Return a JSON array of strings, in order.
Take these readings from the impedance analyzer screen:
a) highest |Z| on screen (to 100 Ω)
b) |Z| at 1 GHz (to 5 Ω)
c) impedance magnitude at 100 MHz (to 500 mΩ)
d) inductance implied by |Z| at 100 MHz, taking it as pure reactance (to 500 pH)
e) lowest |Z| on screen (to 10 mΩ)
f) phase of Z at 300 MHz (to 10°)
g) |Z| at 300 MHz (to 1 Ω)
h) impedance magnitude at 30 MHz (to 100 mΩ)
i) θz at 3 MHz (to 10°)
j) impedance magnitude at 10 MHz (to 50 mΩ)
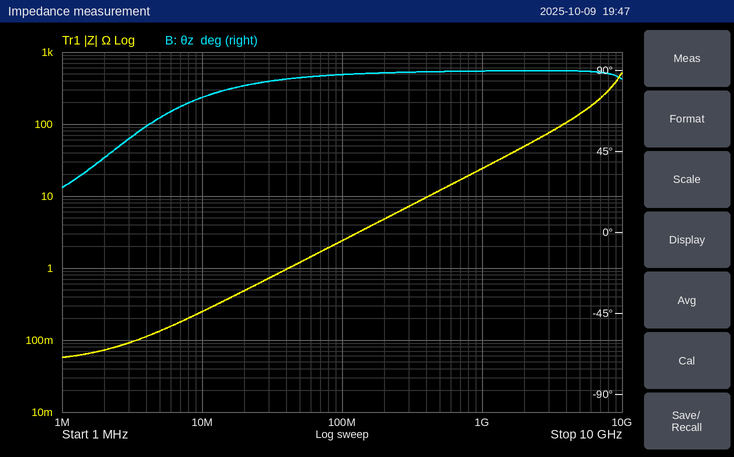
["500 Ω", "25 Ω", "2.5 Ω", "4.0 nH", "60 mΩ", "90°", "7 Ω", "700 mΩ", "50°", "250 mΩ"]
